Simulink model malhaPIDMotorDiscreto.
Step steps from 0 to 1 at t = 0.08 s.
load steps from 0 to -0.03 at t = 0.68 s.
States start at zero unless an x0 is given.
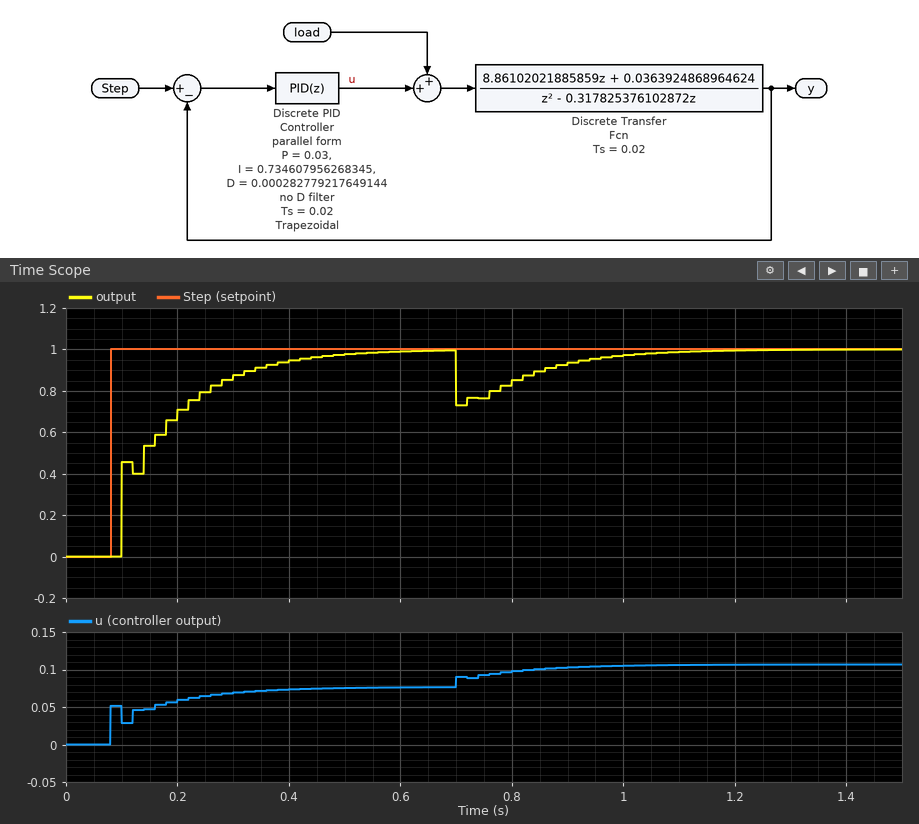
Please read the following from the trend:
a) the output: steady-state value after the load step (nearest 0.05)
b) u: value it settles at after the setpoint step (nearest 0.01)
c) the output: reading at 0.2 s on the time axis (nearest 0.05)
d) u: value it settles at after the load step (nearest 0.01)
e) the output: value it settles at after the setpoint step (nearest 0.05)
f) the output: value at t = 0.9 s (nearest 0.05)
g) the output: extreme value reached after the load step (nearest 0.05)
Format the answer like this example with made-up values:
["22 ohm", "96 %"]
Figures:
["1.00", "0.08", "0.70", "0.11", "1.00", "0.95", "0.75"]
